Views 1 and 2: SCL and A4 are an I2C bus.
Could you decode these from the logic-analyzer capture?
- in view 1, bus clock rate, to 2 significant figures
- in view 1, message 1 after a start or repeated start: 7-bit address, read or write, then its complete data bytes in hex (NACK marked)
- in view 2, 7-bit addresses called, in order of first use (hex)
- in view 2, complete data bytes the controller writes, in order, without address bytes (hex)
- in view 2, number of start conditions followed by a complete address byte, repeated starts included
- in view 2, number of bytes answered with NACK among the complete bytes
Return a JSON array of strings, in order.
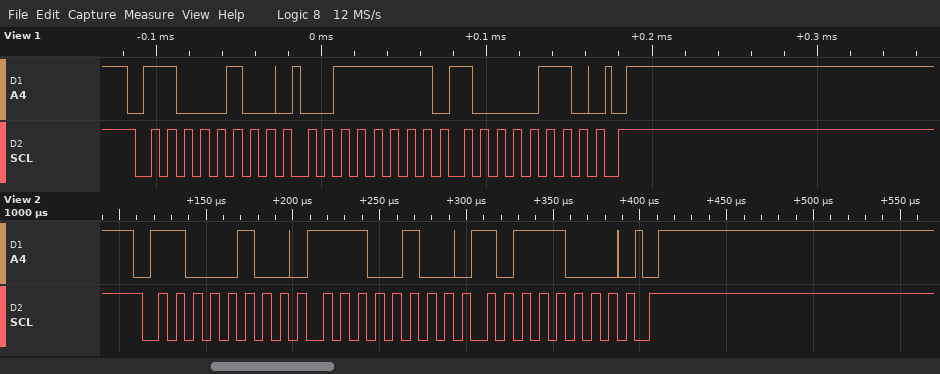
["100 kHz", "0x62 write: 3F 86", "0x62", "E4 B8", "1", "0"]
